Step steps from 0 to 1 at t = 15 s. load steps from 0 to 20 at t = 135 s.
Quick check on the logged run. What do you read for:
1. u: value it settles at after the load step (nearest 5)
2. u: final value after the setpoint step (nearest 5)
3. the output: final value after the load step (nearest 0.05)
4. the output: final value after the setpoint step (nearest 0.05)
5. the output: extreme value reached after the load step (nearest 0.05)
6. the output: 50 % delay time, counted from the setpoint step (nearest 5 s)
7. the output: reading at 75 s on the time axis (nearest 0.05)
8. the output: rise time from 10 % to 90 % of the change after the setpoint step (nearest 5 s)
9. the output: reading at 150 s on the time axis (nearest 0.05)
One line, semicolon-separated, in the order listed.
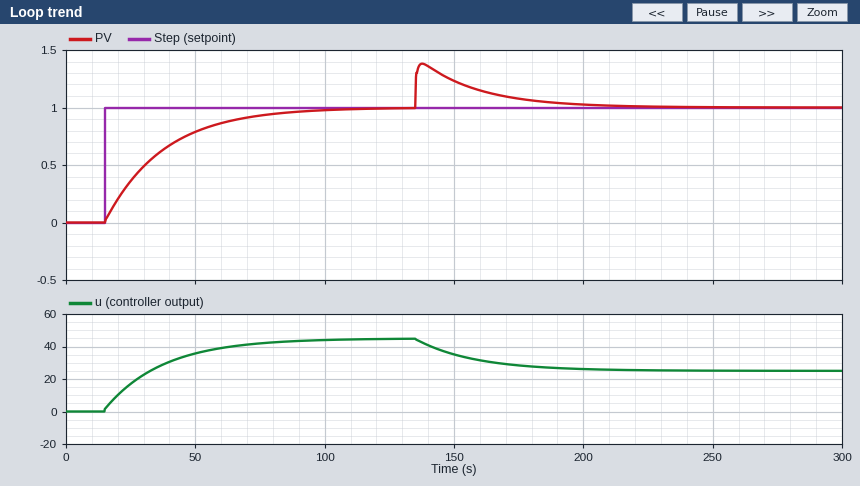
25; 45; 1.00; 1.00; 1.40; 15 s; 0.95; 50 s; 1.25
